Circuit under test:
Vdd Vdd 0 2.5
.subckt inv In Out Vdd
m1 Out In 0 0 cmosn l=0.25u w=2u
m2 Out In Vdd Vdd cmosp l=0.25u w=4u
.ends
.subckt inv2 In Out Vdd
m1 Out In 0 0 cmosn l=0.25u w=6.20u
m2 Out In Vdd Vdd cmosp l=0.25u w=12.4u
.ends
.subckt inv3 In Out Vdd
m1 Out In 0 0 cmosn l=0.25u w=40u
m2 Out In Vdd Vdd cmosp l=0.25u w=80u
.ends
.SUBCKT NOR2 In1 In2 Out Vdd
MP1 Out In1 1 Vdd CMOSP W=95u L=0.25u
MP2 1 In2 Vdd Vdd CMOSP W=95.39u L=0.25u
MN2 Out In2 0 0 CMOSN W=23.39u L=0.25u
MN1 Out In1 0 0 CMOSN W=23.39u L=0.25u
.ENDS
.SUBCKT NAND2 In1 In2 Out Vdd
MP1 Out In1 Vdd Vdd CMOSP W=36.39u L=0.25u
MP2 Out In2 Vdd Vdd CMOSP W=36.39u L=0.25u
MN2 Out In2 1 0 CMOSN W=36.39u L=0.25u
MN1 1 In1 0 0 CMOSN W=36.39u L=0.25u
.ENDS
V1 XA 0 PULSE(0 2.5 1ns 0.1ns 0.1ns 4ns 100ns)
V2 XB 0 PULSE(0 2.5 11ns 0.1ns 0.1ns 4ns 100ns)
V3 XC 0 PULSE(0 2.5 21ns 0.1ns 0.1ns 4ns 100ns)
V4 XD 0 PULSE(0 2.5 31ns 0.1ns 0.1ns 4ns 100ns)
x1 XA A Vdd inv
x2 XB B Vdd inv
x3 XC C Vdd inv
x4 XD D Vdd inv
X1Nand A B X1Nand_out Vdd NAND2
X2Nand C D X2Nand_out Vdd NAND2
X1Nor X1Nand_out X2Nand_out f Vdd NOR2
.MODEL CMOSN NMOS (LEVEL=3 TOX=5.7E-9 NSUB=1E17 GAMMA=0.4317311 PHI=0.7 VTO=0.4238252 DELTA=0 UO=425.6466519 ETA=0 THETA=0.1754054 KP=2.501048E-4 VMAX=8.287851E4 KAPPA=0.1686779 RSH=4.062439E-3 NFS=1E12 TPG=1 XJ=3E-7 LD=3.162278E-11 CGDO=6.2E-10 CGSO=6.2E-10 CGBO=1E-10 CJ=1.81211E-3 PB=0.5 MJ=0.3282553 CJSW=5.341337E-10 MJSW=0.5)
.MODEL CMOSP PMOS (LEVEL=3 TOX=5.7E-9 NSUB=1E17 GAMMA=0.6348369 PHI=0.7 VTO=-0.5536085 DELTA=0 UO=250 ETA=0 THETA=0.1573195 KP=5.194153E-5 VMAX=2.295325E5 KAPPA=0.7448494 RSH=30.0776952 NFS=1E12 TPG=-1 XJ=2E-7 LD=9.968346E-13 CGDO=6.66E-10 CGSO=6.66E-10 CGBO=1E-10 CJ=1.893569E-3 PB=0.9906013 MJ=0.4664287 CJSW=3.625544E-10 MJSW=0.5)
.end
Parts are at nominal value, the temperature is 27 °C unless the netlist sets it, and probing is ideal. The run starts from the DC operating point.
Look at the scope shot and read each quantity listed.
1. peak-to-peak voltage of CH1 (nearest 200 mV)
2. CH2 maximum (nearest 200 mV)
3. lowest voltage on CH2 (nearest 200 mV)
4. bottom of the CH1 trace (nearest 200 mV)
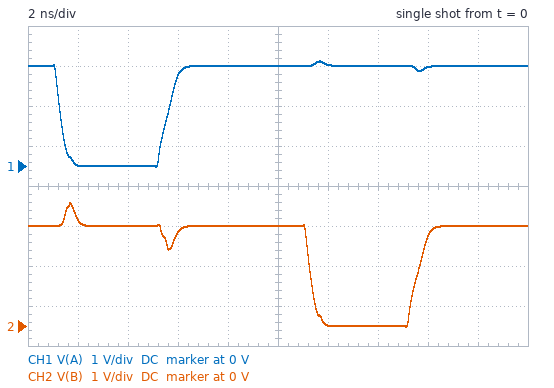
2.6 V
3.0 V
0 V
0 V
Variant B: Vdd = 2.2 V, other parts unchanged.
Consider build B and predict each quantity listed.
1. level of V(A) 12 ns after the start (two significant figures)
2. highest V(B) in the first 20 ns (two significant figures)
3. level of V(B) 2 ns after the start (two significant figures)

2.2 V
2.7 V
2.3 V
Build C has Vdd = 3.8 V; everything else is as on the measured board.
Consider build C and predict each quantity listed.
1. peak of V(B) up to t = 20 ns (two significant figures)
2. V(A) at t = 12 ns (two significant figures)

4.4 V
3.9 V
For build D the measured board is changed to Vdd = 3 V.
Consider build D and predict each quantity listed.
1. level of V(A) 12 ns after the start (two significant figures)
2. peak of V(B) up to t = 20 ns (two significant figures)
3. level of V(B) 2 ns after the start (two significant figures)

3.0 V
3.6 V
3.2 V
